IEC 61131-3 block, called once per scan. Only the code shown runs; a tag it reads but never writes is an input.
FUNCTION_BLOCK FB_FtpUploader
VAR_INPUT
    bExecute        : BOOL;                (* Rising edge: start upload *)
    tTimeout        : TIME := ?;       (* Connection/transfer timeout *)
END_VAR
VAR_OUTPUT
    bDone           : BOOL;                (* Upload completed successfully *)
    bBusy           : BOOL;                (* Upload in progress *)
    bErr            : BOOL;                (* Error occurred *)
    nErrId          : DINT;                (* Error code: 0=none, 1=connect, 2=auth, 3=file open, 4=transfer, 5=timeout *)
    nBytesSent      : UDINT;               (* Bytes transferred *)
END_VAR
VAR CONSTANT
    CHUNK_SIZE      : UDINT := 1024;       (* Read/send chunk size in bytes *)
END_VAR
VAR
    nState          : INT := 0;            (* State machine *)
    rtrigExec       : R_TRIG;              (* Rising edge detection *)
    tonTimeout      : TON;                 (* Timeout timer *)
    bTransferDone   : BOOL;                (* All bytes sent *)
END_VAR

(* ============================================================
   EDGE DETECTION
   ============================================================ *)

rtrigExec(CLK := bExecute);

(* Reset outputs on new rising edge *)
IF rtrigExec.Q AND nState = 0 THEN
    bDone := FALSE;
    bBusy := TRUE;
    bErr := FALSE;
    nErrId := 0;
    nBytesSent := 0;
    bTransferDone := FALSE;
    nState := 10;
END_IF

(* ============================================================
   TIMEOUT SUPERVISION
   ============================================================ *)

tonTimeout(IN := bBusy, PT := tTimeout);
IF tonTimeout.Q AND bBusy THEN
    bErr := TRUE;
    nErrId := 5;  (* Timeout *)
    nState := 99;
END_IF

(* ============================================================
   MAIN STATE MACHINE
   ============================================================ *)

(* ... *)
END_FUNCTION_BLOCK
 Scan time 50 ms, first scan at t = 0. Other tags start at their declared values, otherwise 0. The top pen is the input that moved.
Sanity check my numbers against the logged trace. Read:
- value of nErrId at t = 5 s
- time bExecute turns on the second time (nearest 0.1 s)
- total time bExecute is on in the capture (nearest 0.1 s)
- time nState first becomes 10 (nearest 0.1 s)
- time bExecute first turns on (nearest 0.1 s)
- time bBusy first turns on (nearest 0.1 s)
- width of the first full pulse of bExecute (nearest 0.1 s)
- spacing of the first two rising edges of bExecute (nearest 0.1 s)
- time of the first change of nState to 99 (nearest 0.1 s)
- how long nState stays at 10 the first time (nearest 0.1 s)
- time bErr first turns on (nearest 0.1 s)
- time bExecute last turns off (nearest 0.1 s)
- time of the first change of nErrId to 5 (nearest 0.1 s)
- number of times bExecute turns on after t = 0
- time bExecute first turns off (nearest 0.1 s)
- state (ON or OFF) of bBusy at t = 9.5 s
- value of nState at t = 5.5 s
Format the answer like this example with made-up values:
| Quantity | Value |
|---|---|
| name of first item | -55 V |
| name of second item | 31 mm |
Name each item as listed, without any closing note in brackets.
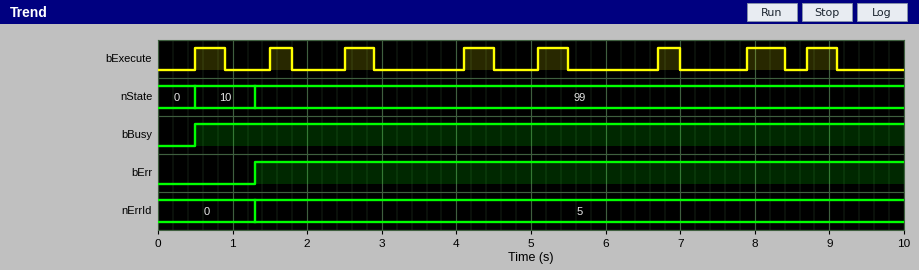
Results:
| Quantity | Value |
|---|---|
| value of nErrId at t = 5 s | 5 |
| time bExecute turns on the second time | 1.5 s |
| total time bExecute is on in the capture | 3.1 s |
| time nState first becomes 10 | 0.5 s |
| time bExecute first turns on | 0.5 s |
| time bBusy first turns on | 0.5 s |
| width of the first full pulse of bExecute | 0.4 s |
| spacing of the first two rising edges of bExecute | 1.0 s |
| time of the first change of nState to 99 | 1.3 s |
| how long nState stays at 10 the first time | 0.8 s |
| time bErr first turns on | 1.3 s |
| time bExecute last turns off | 9.1 s |
| time of the first change of nErrId to 5 | 1.3 s |
| number of times bExecute turns on after t = 0 | 8 |
| time bExecute first turns off | 0.9 s |
| state (ON or OFF) of bBusy at t = 9.5 s | ON |
| value of nState at t = 5.5 s | 99 |
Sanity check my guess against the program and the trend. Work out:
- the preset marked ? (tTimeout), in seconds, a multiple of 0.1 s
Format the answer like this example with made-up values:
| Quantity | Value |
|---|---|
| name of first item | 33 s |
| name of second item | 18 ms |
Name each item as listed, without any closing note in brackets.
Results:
| Quantity | Value |
|---|---|
| the preset marked ? (tTimeout), in seconds, a multiple of 0.1 s | 0.8 s |
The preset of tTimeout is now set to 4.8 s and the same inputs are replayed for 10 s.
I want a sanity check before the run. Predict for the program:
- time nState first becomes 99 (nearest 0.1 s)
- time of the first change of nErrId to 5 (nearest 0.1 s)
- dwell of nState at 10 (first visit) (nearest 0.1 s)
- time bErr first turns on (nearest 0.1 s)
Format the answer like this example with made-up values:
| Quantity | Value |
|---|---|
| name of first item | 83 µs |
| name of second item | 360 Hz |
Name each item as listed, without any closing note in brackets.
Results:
| Quantity | Value |
|---|---|
| time nState first becomes 99 | 5.3 s |
| time of the first change of nErrId to 5 | 5.3 s |
| dwell of nState at 10 (first visit) | 4.8 s |
| time bErr first turns on | 5.3 s |
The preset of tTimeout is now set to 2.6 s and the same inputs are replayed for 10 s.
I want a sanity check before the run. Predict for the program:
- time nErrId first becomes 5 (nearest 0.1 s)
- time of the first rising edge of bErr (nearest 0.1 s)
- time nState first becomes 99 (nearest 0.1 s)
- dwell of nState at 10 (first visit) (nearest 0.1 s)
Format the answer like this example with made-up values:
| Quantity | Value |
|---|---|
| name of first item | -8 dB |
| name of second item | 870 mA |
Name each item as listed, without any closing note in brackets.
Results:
| Quantity | Value |
|---|---|
| time nErrId first becomes 5 | 3.1 s |
| time of the first rising edge of bErr | 3.1 s |
| time nState first becomes 99 | 3.1 s |
| dwell of nState at 10 (first visit) | 2.6 s |
